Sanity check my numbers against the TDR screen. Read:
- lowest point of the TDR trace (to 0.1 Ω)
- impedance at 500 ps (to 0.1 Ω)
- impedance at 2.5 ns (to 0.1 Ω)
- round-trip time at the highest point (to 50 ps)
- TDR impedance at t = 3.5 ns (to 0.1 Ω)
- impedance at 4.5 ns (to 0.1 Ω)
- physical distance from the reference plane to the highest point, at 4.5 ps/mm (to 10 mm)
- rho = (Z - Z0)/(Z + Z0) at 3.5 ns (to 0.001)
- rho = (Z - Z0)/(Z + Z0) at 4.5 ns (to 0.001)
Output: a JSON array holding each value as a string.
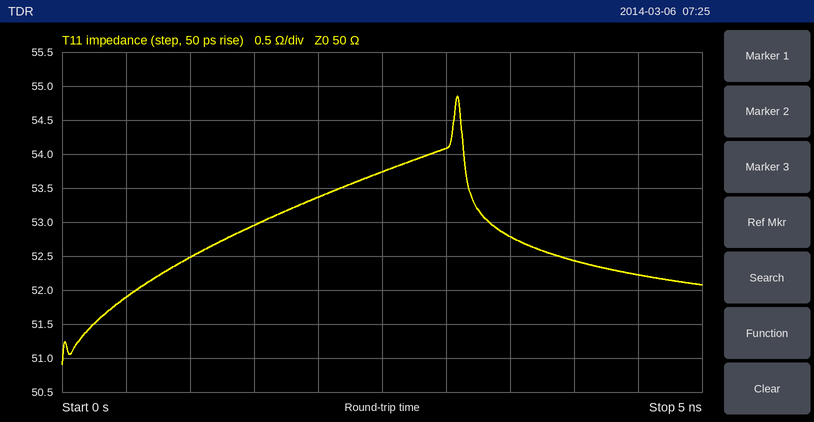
["50.9 Ω", "51.9 Ω", "53.7 Ω", "3.10 ns", "52.8 Ω", "52.2 Ω", "340 mm", "+0.027", "+0.022"]
